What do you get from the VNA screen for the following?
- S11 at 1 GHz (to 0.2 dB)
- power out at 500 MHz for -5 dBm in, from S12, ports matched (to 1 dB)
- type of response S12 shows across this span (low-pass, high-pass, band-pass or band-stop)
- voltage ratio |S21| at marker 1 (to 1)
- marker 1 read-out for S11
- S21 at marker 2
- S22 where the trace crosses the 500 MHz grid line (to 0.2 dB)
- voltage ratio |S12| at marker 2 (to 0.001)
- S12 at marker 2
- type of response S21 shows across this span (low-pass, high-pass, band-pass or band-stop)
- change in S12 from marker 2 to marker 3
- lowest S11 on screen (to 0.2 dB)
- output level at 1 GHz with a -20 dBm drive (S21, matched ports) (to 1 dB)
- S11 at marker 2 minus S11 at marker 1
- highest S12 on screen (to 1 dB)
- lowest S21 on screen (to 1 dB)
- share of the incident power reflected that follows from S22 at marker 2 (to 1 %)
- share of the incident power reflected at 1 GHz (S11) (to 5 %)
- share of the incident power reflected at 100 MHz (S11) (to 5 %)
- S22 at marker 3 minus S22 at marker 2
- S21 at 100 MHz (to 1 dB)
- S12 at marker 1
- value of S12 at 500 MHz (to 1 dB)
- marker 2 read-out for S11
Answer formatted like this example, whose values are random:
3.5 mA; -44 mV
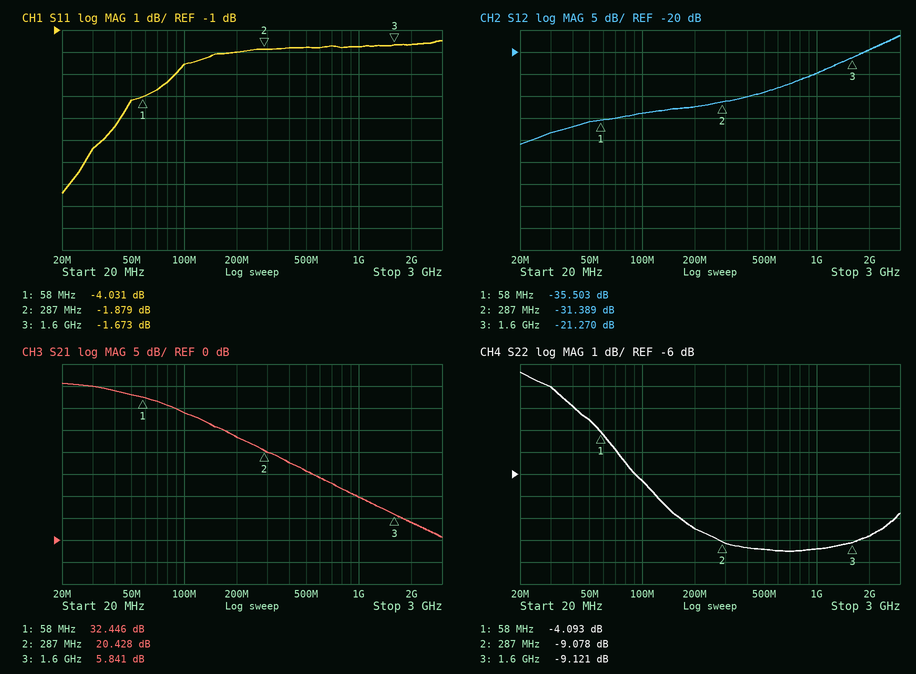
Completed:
-1.8 dB; -34 dBm; high-pass; 42; -4.031 dB; 20.428 dB; -9.4 dB; 0.027; -31.389 dB; low-pass; 10.119 dB; -8.4 dB; -10 dBm; 2.152 dB; -16 dB; 1 dB; 12 %; 65 %; 55 %; -0.043 dB; 29 dB; -35.503 dB; -29 dB; -1.879 dB
